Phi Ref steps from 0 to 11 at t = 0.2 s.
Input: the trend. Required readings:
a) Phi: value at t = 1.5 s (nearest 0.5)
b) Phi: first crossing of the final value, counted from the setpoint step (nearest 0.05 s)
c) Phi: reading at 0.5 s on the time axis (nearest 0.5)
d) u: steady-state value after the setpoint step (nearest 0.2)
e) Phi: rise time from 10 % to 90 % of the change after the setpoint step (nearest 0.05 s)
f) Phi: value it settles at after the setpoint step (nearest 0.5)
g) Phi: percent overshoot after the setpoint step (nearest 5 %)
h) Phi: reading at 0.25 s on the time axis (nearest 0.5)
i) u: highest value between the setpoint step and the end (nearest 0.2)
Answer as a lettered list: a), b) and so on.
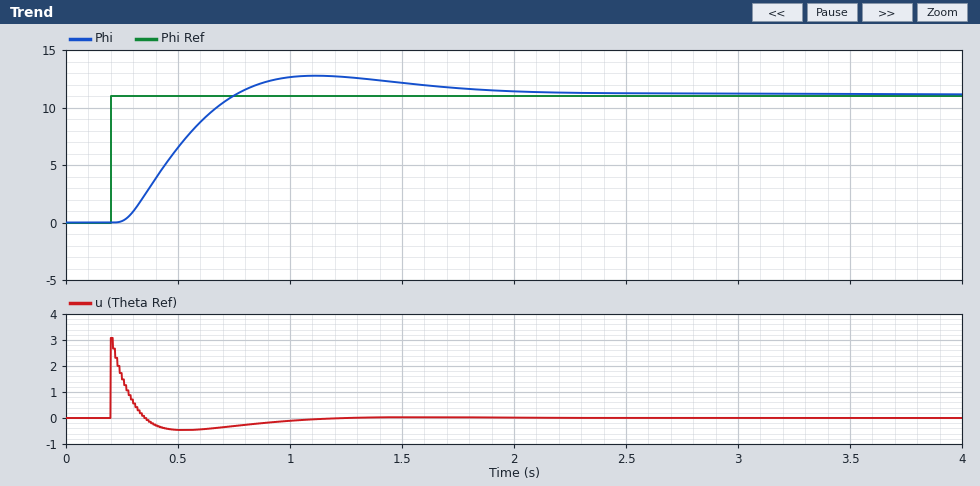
a) 12.0
b) 0.55 s
c) 6.5
d) 0.0
e) 0.35 s
f) 11.0
g) 15 %
h) 0.0
i) 3.0
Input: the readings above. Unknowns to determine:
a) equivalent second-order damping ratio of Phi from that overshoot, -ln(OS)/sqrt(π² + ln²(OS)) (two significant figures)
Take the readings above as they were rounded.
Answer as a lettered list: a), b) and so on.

a) 0.52
